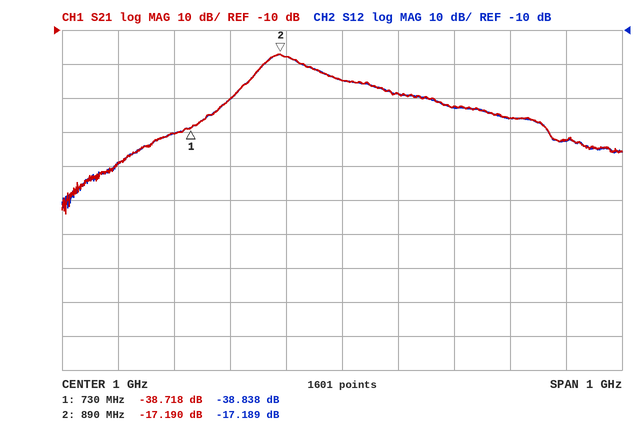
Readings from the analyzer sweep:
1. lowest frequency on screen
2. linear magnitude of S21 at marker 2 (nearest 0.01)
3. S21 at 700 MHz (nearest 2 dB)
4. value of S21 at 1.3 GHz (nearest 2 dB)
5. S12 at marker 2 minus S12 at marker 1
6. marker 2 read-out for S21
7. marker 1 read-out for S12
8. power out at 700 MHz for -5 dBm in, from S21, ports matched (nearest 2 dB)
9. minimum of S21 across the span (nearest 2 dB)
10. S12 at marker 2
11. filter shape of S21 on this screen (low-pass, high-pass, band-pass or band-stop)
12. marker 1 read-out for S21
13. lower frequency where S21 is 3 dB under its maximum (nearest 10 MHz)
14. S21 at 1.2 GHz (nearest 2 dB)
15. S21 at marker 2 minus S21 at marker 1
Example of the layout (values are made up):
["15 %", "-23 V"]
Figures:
["500 MHz", "0.14", "-40 dB", "-36 dB", "21.649 dB", "-17.190 dB", "-38.838 dB", "-46 dBm", "-64 dB", "-17.189 dB", "band-pass", "-38.718 dB", "860 MHz", "-32 dB", "21.528 dB"]
